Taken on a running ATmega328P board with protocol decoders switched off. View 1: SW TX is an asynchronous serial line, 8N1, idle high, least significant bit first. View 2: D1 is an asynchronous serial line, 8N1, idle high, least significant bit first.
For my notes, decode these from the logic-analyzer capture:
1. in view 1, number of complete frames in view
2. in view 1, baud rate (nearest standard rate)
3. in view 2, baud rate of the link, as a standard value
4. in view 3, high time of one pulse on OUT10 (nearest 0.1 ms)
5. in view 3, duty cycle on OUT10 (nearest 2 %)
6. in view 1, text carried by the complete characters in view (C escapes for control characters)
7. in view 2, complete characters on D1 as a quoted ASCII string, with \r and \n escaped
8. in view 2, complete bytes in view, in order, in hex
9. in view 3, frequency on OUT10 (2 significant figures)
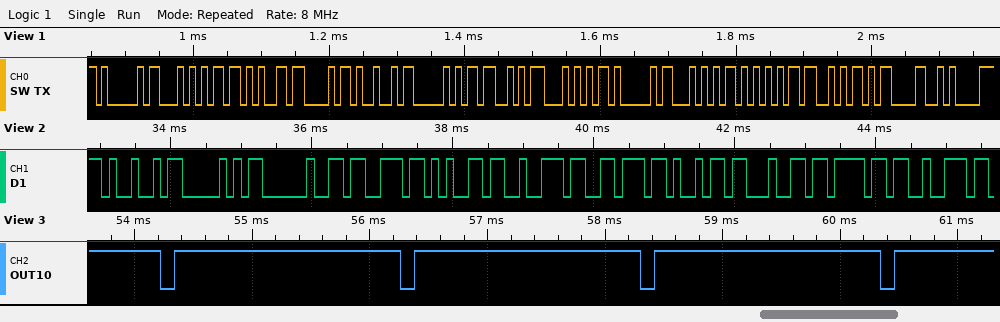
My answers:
14
115200 baud
9600 baud
1.9 ms
94 %
"AT+CIPSTATUS\r\n"
"IP servidor"
49 50 20 73 65 72 76 69 64 6F 72
490 Hz
